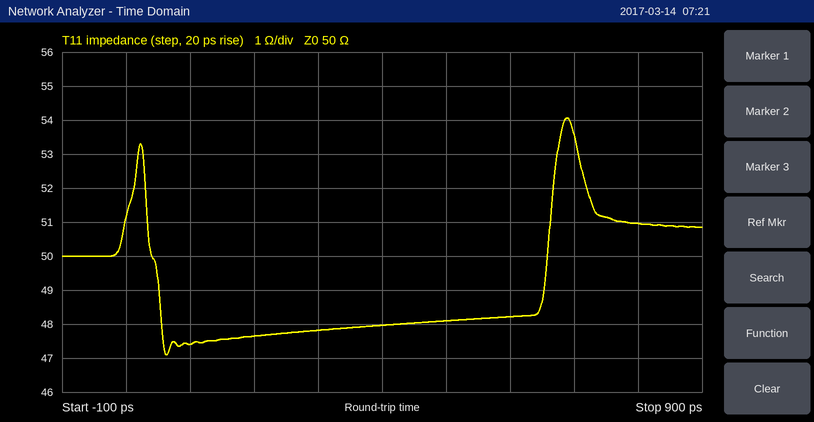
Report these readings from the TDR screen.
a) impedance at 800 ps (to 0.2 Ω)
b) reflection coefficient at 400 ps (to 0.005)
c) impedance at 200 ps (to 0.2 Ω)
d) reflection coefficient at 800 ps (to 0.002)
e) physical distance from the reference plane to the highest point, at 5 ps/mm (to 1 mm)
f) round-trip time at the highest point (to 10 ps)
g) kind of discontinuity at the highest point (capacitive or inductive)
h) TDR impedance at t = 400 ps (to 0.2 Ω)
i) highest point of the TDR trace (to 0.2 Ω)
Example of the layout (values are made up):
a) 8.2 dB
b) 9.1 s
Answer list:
a) 51.0 Ω
b) -0.020
c) 47.6 Ω
d) +0.010
e) 69 mm
f) 690 ps
g) inductive
h) 48.0 Ω
i) 54.0 Ω
